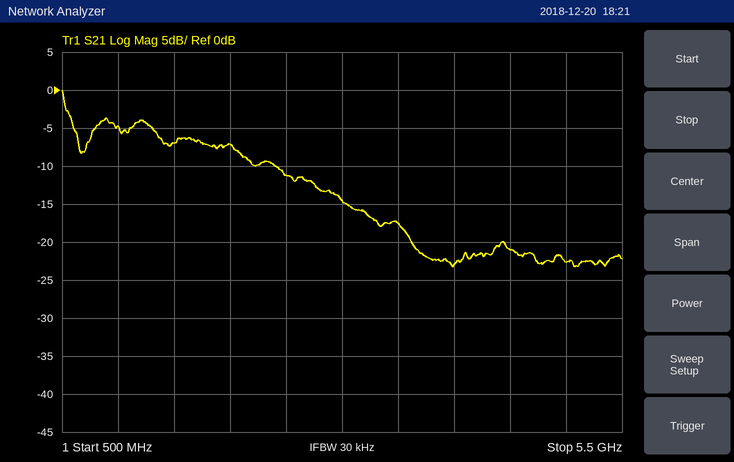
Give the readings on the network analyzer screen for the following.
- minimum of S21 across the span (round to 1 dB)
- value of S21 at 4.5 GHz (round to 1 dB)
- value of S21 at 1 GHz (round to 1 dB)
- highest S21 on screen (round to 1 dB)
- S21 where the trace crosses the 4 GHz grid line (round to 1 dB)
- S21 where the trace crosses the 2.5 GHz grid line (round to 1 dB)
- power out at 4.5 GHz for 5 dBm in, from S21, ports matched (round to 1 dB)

-23 dB
-21 dB
-5 dB
0 dB
-23 dB
-11 dB
-16 dBm
